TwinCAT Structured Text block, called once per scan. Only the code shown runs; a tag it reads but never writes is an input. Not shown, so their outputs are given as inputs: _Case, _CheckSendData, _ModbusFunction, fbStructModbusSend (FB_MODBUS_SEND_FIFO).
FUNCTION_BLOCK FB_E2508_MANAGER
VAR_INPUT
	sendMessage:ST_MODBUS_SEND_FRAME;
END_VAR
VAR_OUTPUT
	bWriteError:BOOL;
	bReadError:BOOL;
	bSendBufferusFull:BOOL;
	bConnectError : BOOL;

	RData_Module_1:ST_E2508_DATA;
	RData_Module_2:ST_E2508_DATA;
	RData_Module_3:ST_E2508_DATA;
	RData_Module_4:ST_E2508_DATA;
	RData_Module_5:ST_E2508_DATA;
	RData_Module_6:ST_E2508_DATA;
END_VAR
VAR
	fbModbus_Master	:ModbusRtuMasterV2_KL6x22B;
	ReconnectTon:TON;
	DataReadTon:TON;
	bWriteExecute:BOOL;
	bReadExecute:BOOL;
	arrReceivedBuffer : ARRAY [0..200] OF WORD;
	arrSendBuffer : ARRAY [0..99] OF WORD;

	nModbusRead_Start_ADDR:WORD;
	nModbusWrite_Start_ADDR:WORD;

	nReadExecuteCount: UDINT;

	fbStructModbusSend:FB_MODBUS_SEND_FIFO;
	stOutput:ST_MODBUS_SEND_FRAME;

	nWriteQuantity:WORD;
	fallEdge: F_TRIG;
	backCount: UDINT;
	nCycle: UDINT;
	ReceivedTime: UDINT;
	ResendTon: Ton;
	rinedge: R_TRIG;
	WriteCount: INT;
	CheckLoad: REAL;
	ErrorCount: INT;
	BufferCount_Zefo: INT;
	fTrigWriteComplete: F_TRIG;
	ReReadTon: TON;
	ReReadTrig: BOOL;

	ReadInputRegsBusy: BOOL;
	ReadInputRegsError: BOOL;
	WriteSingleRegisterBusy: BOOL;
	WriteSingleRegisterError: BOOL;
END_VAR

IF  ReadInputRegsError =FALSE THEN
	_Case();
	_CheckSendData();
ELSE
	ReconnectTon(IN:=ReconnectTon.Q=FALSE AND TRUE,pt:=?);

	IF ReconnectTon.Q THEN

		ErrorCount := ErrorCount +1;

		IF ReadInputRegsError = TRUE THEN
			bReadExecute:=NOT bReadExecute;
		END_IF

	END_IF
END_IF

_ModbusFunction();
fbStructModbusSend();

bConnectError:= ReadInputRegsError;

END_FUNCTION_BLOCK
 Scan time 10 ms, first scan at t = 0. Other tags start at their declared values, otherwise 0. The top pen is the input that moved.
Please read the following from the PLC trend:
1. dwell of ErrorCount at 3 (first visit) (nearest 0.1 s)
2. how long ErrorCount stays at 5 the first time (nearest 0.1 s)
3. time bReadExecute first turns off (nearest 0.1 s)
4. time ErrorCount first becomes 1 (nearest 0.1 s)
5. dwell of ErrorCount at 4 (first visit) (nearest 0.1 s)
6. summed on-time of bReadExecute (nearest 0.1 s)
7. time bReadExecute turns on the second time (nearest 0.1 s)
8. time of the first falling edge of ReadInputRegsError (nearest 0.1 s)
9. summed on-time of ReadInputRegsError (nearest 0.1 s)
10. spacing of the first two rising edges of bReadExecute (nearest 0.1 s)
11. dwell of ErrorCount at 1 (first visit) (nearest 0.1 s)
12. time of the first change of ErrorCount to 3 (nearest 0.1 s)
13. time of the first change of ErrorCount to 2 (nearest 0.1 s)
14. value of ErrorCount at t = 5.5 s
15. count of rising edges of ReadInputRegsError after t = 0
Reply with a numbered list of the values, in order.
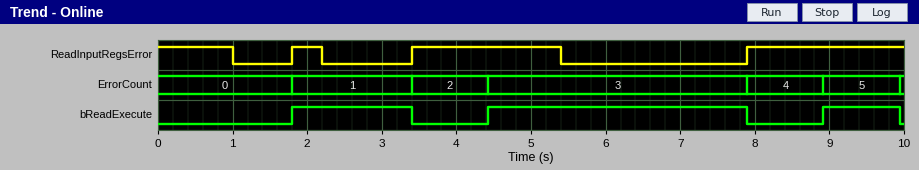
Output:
1. 3.5 s
2. 1.0 s
3. 3.4 s
4. 1.8 s
5. 1.0 s
6. 6.1 s
7. 4.4 s
8. 1.0 s
9. 5.5 s
10. 2.6 s
11. 1.6 s
12. 4.4 s
13. 3.4 s
14. 3
15. 3
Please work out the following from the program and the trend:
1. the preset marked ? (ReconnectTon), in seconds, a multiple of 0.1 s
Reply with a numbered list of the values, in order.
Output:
1. 1.0 s
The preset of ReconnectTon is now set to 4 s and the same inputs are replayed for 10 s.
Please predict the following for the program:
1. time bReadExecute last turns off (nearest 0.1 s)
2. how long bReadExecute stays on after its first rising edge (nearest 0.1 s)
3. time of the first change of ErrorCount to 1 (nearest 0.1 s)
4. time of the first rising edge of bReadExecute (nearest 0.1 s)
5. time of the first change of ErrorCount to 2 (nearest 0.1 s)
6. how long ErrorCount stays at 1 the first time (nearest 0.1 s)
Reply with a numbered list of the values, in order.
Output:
1. 8.0 s
2. 4.0 s
3. 4.0 s
4. 4.0 s
5. 8.0 s
6. 4.0 s
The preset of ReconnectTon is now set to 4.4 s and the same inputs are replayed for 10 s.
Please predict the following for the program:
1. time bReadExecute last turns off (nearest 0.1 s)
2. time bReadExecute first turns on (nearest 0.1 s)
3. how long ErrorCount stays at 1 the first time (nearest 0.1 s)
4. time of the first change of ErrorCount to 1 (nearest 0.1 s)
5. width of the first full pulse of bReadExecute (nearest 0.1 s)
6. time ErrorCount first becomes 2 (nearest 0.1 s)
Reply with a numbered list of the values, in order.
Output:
1. 8.8 s
2. 4.4 s
3. 4.4 s
4. 4.4 s
5. 4.4 s
6. 8.8 s
